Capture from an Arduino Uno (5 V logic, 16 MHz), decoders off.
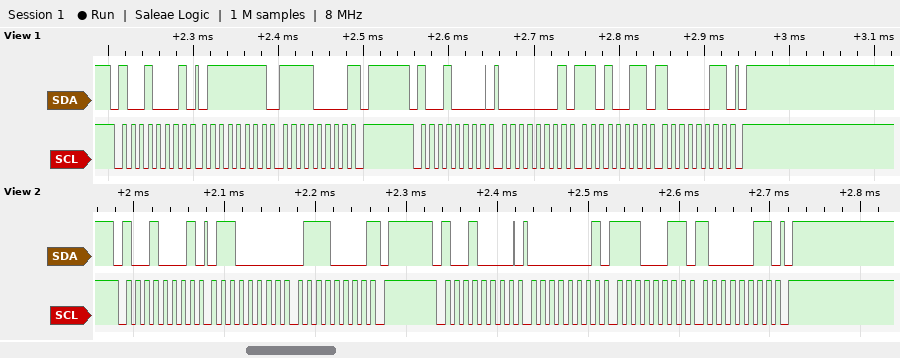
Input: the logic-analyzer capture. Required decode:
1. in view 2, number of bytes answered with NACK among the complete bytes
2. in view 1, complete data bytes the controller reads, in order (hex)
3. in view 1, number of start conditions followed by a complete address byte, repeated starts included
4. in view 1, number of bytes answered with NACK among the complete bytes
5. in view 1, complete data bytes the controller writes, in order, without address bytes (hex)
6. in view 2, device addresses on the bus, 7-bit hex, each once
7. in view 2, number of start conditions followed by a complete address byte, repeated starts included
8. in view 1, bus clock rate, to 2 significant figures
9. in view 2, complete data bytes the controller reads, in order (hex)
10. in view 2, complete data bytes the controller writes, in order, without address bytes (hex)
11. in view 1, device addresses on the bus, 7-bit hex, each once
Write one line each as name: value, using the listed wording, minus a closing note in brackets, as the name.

in view 2, number of bytes answered with NACK among the complete bytes: 1
in view 1, complete data bytes the controller reads, in order: 7F F0
in view 1, number of start conditions followed by a complete address byte, repeated starts included: 2
in view 1, number of bytes answered with NACK among the complete bytes: 1
in view 1, complete data bytes the controller writes, in order, without address bytes: 01 D3 83
in view 2, device addresses on the bus, 7-bit hex, each once: 0x48
in view 2, number of start conditions followed by a complete address byte, repeated starts included: 2
in view 1, bus clock rate, to 2 significant figures: 100 kHz
in view 2, complete data bytes the controller reads, in order: 60 70
in view 2, complete data bytes the controller writes, in order, without address bytes: 01 E3 83
in view 1, device addresses on the bus, 7-bit hex, each once: 0x48
